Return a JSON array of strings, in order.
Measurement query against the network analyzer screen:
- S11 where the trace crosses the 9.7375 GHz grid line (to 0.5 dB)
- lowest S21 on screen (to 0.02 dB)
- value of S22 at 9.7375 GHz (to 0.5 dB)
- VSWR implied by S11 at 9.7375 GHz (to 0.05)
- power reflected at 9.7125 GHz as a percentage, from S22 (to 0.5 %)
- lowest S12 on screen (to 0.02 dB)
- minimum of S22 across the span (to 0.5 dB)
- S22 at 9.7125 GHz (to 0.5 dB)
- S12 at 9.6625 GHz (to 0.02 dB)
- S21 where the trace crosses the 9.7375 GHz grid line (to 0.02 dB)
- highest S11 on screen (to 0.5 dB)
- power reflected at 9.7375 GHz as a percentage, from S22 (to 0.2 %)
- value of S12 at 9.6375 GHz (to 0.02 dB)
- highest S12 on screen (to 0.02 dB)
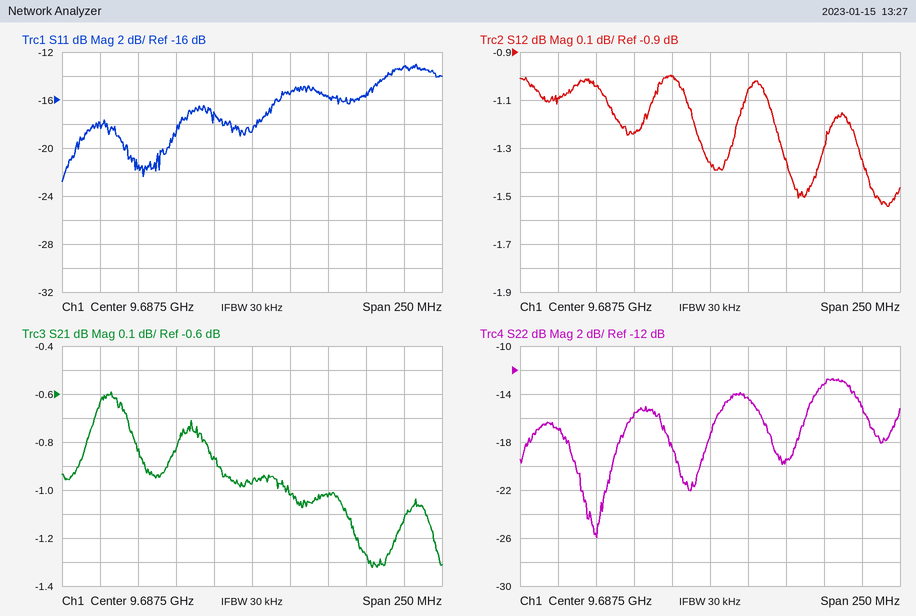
["-15.5 dB", "-1.32 dB", "-19.5 dB", "1.40", "3.5 %", "-1.54 dB", "-26.0 dB", "-14.5 dB", "-1.00 dB", "-1.02 dB", "-13.0 dB", "1.2 %", "-1.24 dB", "-1.00 dB"]
